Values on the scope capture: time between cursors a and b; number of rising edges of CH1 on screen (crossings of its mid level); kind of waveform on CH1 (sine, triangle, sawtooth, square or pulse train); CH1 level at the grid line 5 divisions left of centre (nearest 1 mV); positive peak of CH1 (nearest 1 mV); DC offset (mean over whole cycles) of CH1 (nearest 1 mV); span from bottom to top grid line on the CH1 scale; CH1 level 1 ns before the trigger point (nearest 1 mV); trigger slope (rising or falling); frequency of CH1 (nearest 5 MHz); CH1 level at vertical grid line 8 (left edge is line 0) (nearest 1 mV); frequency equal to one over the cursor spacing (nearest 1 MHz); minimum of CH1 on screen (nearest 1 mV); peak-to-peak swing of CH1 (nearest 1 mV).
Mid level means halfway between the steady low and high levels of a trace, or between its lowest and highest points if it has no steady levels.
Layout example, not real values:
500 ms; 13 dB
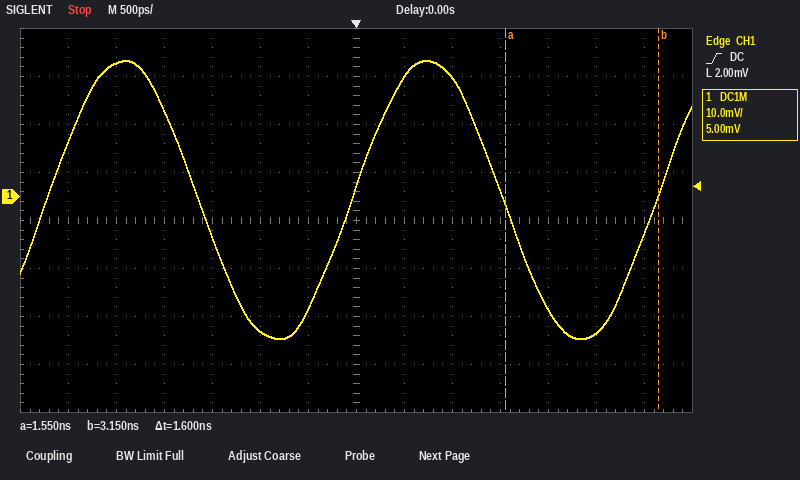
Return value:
1.6 ns; 3; sine; 28 mV; 28 mV; -1 mV; 80 mV; -28 mV; rising; 315 MHz; 25 mV; 625 MHz; -30 mV; 58 mV
